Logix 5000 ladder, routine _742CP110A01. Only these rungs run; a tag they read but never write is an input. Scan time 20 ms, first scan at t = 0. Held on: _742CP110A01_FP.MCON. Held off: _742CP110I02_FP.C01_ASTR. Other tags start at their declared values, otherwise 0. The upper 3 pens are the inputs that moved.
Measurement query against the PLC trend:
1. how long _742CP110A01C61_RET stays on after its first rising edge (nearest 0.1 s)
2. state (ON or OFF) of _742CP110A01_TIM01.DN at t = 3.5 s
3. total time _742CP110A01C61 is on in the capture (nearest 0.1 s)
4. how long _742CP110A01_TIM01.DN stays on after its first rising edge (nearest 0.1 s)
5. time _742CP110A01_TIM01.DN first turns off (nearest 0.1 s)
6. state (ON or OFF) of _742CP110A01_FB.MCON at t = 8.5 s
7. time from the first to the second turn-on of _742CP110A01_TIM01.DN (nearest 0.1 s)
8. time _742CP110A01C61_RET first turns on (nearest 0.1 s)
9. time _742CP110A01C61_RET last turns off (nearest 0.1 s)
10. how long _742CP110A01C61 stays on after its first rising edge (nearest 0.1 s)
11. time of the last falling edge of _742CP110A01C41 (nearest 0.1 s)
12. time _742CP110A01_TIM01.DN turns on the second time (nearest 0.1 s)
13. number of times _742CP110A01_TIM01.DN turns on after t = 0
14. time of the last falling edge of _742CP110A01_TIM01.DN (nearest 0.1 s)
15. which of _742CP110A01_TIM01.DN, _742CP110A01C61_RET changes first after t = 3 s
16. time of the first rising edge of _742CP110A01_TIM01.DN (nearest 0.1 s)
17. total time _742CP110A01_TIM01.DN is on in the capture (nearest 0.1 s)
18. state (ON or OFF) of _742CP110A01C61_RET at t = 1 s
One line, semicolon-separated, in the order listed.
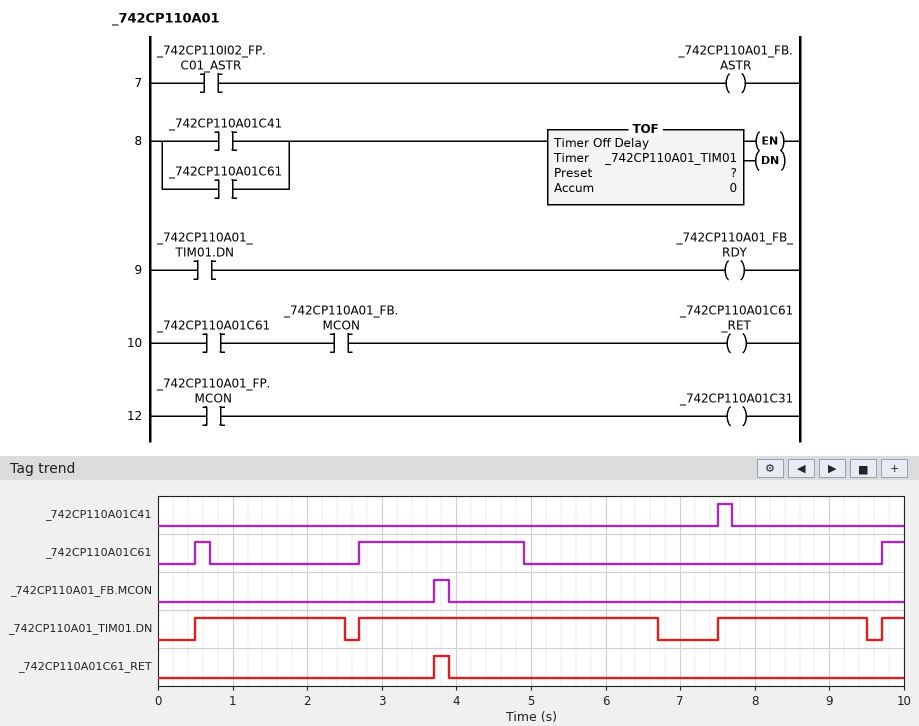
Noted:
0.2 s; ON; 2.7 s; 2.0 s; 2.5 s; OFF; 2.2 s; 3.7 s; 3.9 s; 0.2 s; 7.7 s; 2.7 s; 4; 9.5 s; _742CP110A01C61_RET; 0.5 s; 8.3 s; OFF
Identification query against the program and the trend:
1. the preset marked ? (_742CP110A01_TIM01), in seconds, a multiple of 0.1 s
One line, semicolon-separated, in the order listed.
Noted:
1.8 s
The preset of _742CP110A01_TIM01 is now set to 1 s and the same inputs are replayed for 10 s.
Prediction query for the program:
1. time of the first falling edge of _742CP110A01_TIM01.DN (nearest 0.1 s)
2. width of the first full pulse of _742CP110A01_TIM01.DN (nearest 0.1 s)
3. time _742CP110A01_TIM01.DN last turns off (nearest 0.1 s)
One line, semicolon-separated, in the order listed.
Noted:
1.7 s; 1.2 s; 8.7 s
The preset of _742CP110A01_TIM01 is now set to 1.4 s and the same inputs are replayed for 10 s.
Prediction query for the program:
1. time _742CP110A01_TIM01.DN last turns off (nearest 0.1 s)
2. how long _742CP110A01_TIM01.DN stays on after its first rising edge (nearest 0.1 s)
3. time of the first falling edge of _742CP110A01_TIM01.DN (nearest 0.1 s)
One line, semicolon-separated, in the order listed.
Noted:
9.1 s; 1.6 s; 2.1 s
